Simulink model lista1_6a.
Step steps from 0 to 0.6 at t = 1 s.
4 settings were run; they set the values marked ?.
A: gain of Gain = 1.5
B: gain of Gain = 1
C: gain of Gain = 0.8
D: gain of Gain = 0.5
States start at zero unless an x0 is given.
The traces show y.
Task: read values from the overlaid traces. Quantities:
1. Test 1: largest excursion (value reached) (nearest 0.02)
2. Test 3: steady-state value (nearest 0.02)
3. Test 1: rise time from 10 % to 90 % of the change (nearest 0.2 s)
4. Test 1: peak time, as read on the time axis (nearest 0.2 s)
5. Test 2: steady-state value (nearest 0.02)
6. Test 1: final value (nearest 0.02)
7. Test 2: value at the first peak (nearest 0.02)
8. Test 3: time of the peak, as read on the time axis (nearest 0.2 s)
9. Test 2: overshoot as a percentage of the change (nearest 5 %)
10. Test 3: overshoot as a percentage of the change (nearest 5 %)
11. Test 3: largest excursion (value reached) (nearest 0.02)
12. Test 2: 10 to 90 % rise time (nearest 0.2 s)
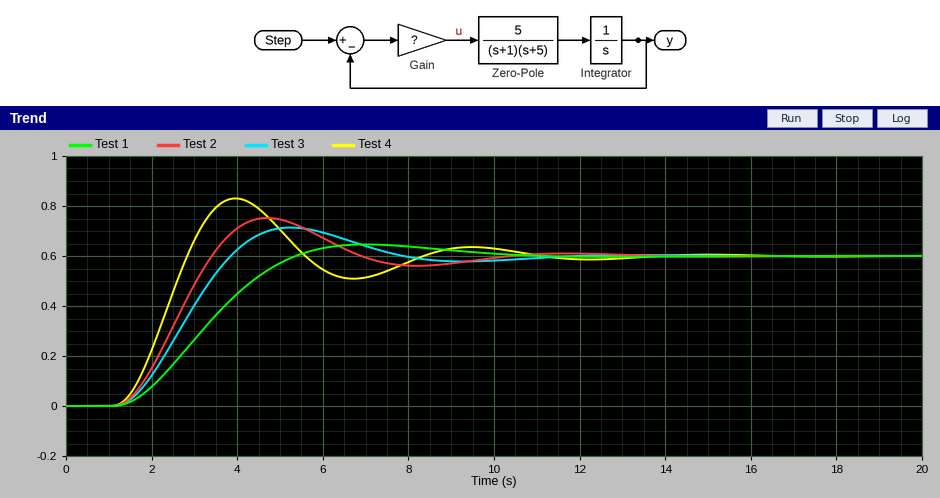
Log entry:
0.64
0.60
2.8 s
7.0 s
0.60
0.60
0.76
5.2 s
25 %
20 %
0.72
1.6 s
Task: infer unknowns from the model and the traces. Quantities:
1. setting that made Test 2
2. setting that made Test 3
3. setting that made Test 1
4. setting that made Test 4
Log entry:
B
C
D
A
